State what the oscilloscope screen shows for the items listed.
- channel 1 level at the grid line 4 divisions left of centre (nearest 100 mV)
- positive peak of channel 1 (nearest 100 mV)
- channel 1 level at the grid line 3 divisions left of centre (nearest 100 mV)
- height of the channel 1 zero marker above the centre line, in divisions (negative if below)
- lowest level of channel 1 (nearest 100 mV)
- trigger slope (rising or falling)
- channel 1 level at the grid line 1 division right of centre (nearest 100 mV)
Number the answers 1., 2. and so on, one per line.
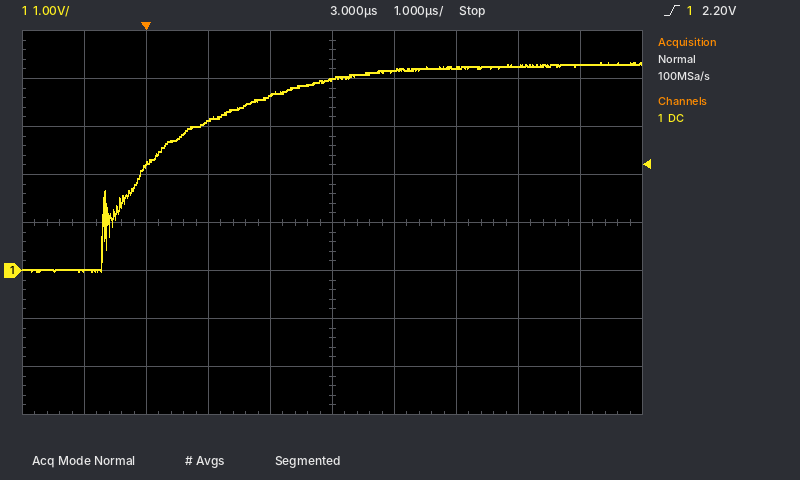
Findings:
1. 0.0 V
2. 4.3 V
3. 2.2 V
4. -1.0 div
5. 0.0 V
6. rising
7. 4.2 V
